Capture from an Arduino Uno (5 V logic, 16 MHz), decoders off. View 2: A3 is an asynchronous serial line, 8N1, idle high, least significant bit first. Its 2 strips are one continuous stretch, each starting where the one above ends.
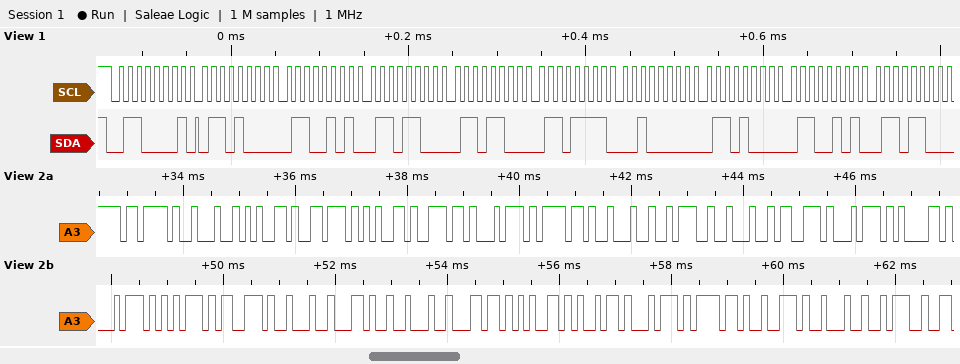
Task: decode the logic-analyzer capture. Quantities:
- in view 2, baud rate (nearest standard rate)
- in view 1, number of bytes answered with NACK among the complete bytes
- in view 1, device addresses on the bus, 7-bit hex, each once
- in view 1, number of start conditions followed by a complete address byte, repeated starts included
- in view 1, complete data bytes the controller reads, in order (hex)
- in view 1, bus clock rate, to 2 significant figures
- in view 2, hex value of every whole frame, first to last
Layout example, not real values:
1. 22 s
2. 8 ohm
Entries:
1. 9600 baud
2. 0
3. 0x30
4. 1
5. 68 65 6C 6C 6F 20 68 65 6C
6. 100 kHz
7. 7B 22 65 76 65 6E 74 6F 22 3A 22 73 74 61 74 75 73 22 2C 22 6C 65 69 74 6F 72 22 3A
